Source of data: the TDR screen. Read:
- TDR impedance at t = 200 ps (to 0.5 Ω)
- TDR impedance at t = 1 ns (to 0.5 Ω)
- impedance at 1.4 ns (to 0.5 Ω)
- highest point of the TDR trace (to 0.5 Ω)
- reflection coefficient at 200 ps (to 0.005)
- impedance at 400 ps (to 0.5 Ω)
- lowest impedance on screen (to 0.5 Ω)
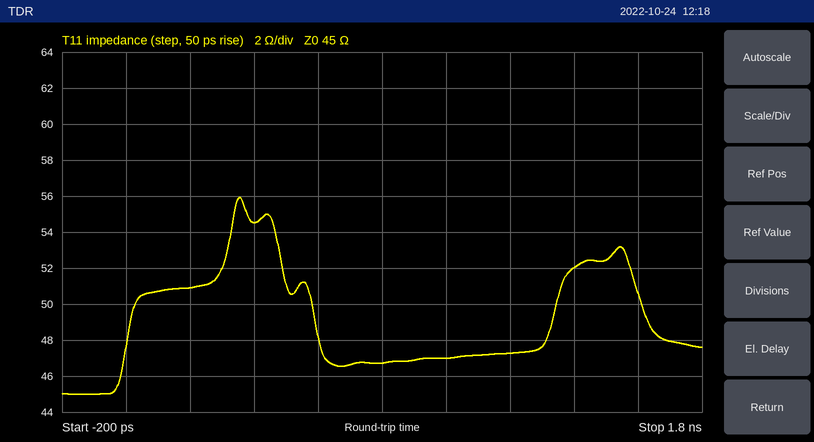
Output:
51.0 Ω
47.0 Ω
52.0 Ω
56.0 Ω
+0.060
54.5 Ω
45.0 Ω
